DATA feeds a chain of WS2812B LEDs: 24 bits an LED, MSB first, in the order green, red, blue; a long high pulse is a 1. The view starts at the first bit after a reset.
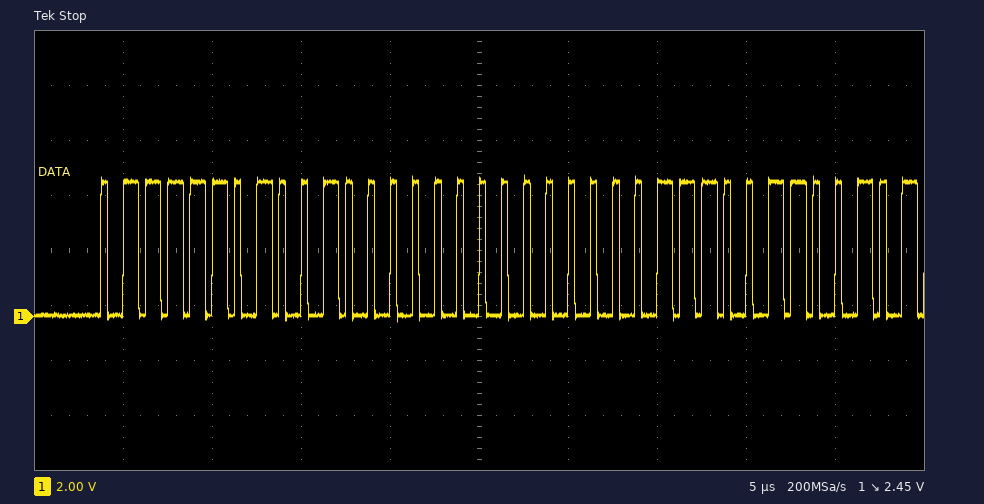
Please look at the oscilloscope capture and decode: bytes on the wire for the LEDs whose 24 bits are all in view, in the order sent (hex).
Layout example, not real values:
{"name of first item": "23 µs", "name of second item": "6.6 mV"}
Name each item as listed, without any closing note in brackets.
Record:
{"bytes on the wire for the LEDs whose 24 bits are all in view, in the order sent": "7D 20 00"}
